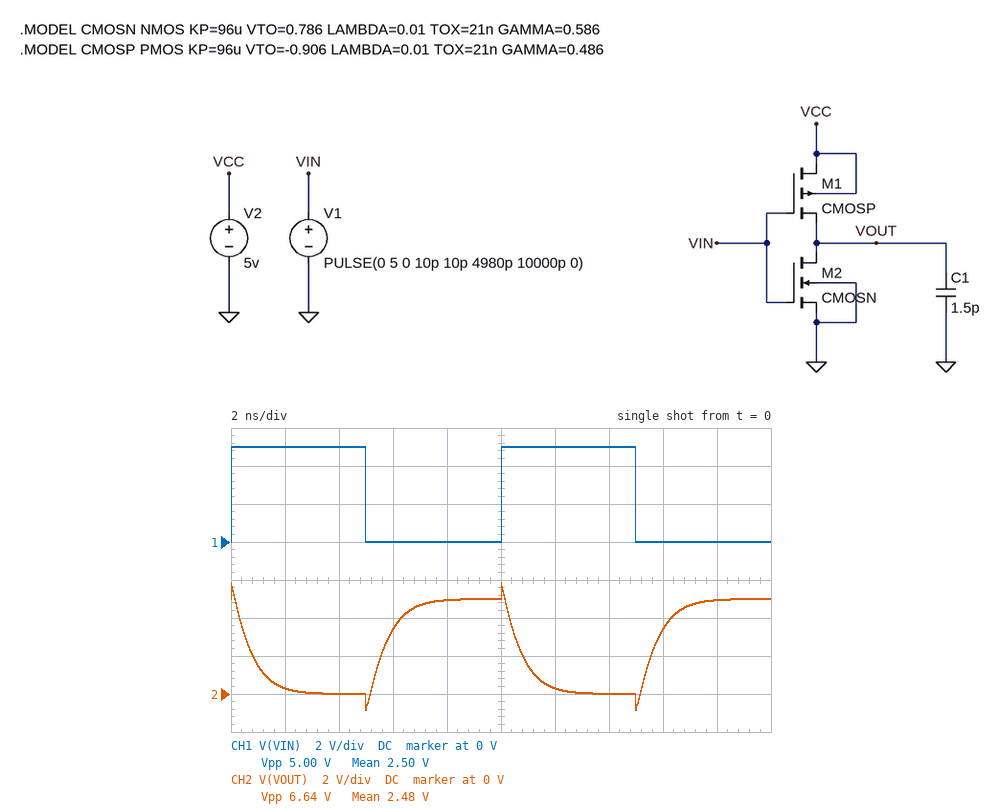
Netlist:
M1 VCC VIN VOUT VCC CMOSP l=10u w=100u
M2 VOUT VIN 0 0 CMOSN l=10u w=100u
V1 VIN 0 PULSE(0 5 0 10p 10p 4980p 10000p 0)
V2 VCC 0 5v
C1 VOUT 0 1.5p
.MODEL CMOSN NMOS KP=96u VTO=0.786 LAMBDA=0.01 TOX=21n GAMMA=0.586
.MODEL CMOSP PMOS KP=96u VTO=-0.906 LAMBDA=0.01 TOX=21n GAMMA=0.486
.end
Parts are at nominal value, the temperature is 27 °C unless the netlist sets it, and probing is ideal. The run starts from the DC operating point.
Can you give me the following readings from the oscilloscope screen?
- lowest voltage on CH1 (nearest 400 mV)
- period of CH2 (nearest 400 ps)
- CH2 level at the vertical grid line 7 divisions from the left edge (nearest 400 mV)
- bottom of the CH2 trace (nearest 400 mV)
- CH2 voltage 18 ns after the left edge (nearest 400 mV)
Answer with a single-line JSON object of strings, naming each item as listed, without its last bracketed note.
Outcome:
{"lowest voltage on CH1": "0 V", "period of CH2": "10.0 ns", "CH2 level at the vertical grid line 7 divisions from the left edge": "0 V", "bottom of the CH2 trace": "-800 mV", "CH2 voltage 18 ns after the left edge": "4.8 V"}
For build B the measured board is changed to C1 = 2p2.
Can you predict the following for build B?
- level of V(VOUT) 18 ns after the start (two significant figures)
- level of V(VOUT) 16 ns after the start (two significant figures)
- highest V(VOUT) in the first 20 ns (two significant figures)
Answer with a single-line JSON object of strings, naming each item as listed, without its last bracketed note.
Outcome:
{"level of V(VOUT) 18 ns after the start": "4.8 V", "level of V(VOUT) 16 ns after the start": "2.6 V", "highest V(VOUT) in the first 20 ns": "5.8 V"}
